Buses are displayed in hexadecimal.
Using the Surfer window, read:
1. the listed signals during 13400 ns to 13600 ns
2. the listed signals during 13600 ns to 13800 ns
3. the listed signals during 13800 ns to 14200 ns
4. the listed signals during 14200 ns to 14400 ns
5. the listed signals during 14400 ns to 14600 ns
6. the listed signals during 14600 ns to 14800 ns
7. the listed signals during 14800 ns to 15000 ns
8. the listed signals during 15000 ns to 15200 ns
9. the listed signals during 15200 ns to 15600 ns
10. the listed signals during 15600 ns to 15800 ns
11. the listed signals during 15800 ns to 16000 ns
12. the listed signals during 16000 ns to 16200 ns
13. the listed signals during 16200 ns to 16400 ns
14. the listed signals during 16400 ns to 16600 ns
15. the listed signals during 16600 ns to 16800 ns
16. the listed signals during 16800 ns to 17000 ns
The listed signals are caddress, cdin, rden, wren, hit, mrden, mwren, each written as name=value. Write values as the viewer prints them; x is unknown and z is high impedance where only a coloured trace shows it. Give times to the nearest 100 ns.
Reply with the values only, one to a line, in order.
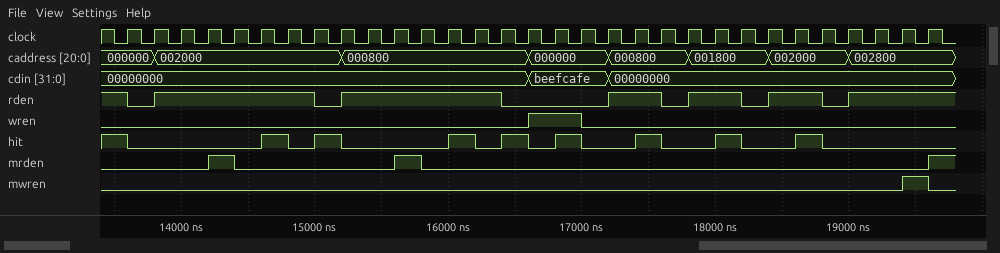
caddress=000000, cdin=00000000, rden=1, wren=0, hit=1, mrden=0, mwren=0
caddress=000000, cdin=00000000, rden=0, wren=0, hit=0, mrden=0, mwren=0
caddress=002000, cdin=00000000, rden=1, wren=0, hit=0, mrden=0, mwren=0
caddress=002000, cdin=00000000, rden=1, wren=0, hit=0, mrden=1, mwren=0
caddress=002000, cdin=00000000, rden=1, wren=0, hit=0, mrden=0, mwren=0
caddress=002000, cdin=00000000, rden=1, wren=0, hit=1, mrden=0, mwren=0
caddress=002000, cdin=00000000, rden=1, wren=0, hit=0, mrden=0, mwren=0
caddress=002000, cdin=00000000, rden=0, wren=0, hit=1, mrden=0, mwren=0
caddress=000800, cdin=00000000, rden=1, wren=0, hit=0, mrden=0, mwren=0
caddress=000800, cdin=00000000, rden=1, wren=0, hit=0, mrden=1, mwren=0
caddress=000800, cdin=00000000, rden=1, wren=0, hit=0, mrden=0, mwren=0
caddress=000800, cdin=00000000, rden=1, wren=0, hit=1, mrden=0, mwren=0
caddress=000800, cdin=00000000, rden=1, wren=0, hit=0, mrden=0, mwren=0
caddress=000800, cdin=00000000, rden=0, wren=0, hit=1, mrden=0, mwren=0
caddress=000000, cdin=beefcafe, rden=0, wren=1, hit=0, mrden=0, mwren=0
caddress=000000, cdin=beefcafe, rden=0, wren=1, hit=1, mrden=0, mwren=0
